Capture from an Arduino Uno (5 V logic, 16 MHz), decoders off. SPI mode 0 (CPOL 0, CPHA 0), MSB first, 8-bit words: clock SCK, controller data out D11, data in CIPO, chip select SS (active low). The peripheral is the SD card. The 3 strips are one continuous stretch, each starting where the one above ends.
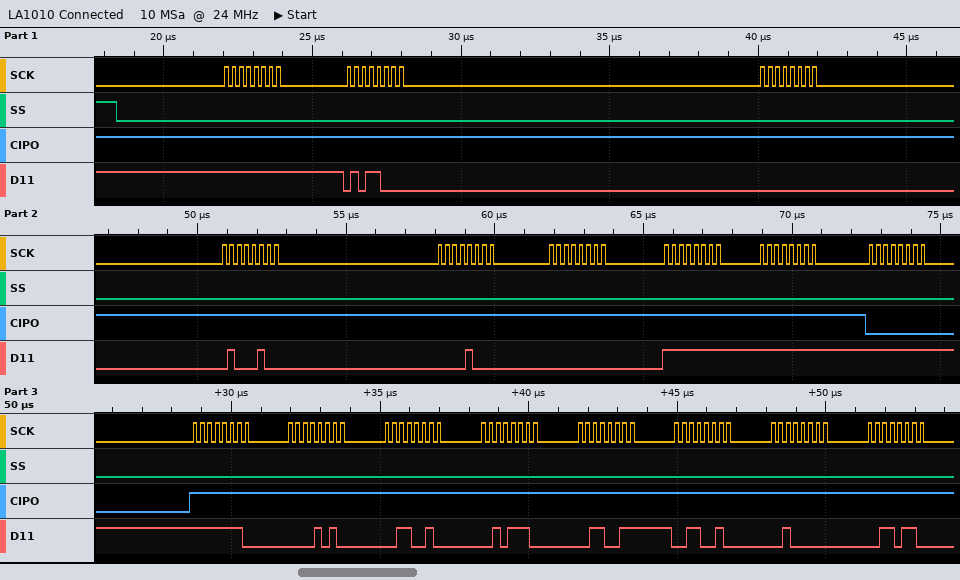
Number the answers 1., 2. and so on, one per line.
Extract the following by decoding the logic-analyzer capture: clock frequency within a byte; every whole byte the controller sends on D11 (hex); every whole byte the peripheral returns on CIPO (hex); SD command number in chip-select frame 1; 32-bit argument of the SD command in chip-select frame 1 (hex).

1. 4 MHz
2. FF 58 00 44 08 00 FF FF FF FE 0A 32 2E 33 32 20 36
3. FF FF FF FF FF FF FF FF 00 FF FF FF FF FF FF FF FF
4. CMD24
5. 0x00440800
